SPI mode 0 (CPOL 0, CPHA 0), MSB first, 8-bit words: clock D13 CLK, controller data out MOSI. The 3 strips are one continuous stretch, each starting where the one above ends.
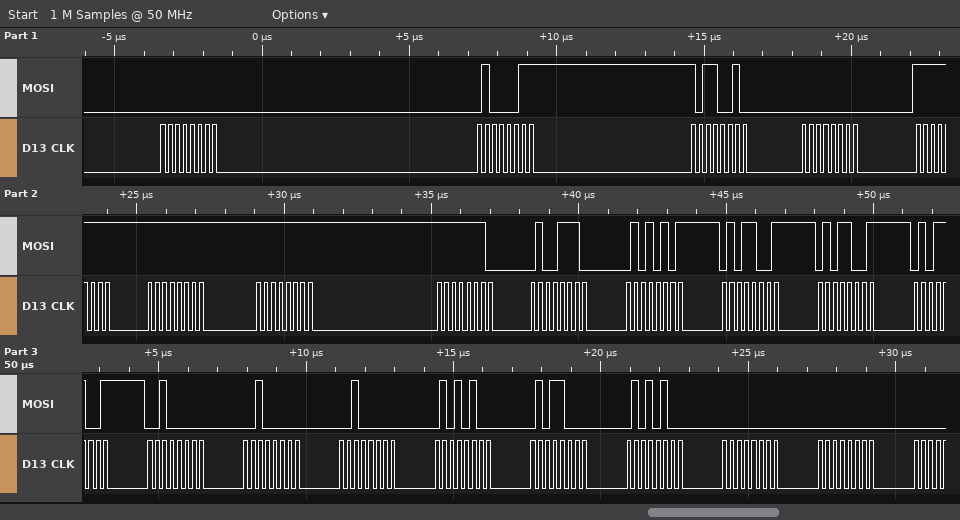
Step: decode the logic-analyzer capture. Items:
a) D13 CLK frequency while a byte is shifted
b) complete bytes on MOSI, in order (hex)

4 MHz
00 43 B2 00 FF FF FF FE 4E 55 59 59 59 20 20 20 54 58 54 00 00
